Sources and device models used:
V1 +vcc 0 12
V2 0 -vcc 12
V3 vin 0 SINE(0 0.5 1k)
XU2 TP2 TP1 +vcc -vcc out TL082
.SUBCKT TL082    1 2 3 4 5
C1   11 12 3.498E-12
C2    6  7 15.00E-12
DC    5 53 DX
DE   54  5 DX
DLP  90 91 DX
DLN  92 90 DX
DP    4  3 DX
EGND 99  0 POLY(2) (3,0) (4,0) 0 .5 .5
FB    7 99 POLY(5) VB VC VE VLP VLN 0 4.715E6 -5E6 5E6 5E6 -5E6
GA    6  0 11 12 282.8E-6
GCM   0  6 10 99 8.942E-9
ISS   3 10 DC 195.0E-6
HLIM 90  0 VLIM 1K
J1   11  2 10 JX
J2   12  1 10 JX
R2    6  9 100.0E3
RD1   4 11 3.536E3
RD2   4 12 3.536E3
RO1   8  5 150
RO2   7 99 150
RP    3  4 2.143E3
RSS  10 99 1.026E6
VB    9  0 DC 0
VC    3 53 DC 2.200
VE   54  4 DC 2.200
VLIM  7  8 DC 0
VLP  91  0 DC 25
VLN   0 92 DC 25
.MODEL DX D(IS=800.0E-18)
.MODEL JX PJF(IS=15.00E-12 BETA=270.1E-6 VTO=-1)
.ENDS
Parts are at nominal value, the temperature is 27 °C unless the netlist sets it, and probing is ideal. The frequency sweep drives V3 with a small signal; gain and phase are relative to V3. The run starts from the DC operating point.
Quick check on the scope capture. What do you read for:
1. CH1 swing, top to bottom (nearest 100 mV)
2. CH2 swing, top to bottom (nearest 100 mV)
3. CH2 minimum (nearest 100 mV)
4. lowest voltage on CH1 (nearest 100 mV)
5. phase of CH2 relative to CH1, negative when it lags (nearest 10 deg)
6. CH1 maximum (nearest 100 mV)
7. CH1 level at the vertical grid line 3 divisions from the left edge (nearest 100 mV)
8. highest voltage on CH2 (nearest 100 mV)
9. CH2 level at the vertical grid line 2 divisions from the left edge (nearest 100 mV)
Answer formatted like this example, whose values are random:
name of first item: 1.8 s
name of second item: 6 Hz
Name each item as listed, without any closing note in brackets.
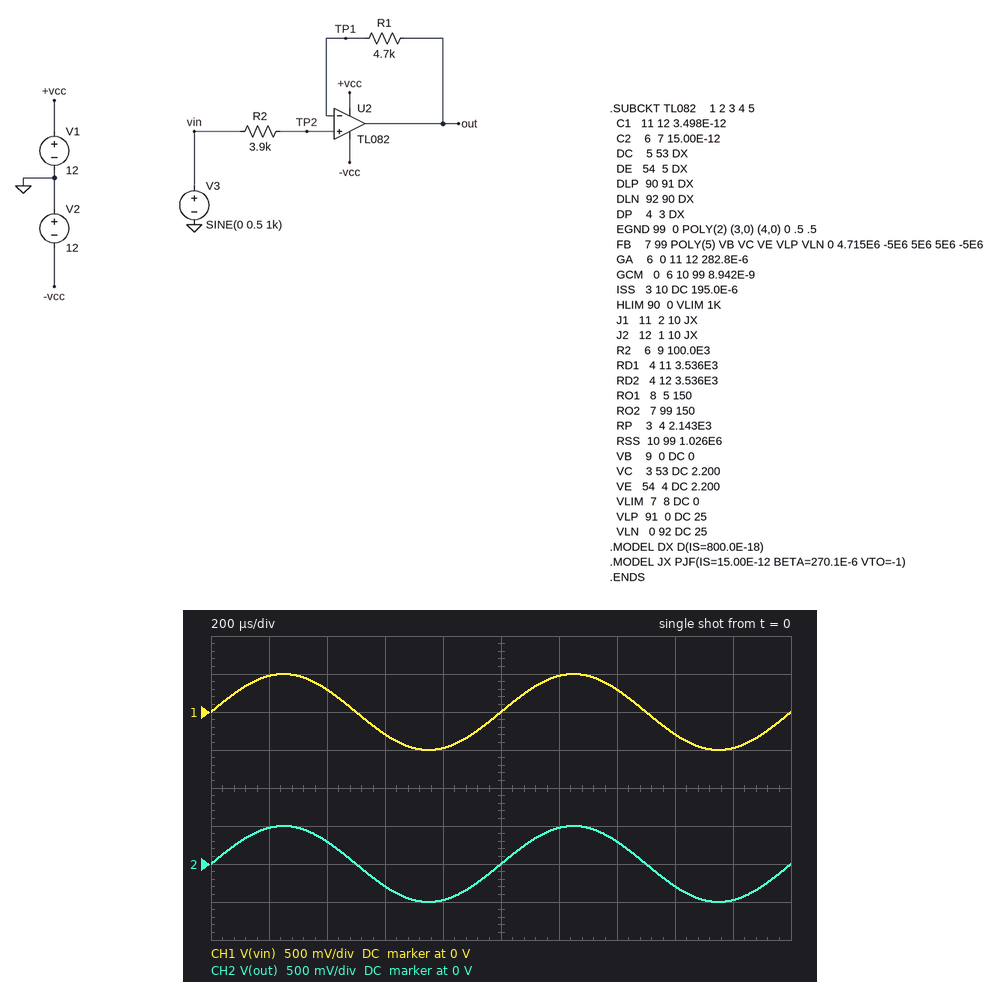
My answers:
CH1 swing, top to bottom: 1.0 V
CH2 swing, top to bottom: 1.0 V
CH2 minimum: -500 mV
lowest voltage on CH1: -500 mV
phase of CH2 relative to CH1, negative when it lags: 0 deg
CH1 maximum: 500 mV
CH1 level at the vertical grid line 3 divisions from the left edge: -300 mV
highest voltage on CH2: 500 mV
CH2 level at the vertical grid line 2 divisions from the left edge: 300 mV
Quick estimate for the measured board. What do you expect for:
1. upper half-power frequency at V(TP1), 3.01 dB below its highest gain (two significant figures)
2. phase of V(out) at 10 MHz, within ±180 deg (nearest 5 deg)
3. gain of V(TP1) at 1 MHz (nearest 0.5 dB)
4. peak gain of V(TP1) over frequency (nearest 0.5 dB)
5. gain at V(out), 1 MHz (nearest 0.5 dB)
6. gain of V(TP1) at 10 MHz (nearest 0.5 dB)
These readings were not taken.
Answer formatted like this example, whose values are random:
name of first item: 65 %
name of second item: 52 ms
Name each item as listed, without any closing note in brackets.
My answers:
upper half-power frequency at V(TP1), 3.01 dB below its highest gain: 4.9 MHz
phase of V(out) at 10 MHz, within ±180 deg: -140 deg
gain of V(TP1) at 1 MHz: 0 dB
peak gain of V(TP1) over frequency: 0 dB
gain at V(out), 1 MHz: 0 dB
gain of V(TP1) at 10 MHz: -13.0 dB
